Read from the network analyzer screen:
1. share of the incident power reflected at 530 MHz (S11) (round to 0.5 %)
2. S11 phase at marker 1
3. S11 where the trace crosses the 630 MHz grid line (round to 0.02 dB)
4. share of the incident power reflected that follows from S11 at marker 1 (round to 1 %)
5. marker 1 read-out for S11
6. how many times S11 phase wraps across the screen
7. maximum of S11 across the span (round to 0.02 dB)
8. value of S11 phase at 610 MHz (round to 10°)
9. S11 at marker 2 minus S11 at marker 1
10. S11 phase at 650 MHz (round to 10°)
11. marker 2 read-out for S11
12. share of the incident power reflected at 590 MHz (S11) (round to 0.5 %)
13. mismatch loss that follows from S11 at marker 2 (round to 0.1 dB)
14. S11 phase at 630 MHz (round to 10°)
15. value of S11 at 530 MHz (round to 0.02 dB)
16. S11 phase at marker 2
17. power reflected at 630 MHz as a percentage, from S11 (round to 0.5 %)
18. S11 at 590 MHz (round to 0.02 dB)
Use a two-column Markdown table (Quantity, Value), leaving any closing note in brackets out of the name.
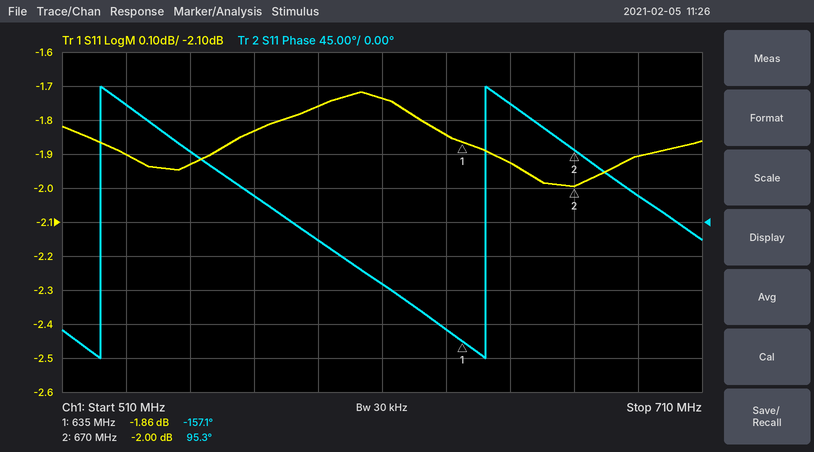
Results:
| Quantity | Value |
|---|---|
| share of the incident power reflected at 530 MHz (S11) | 64.5 % |
| S11 phase at marker 1 | -157.1° |
| S11 where the trace crosses the 630 MHz grid line | -1.84 dB |
| share of the incident power reflected that follows from S11 at marker 1 | 65 % |
| marker 1 read-out for S11 | -1.86 dB |
| how many times S11 phase wraps across the screen | 2 |
| maximum of S11 across the span | -1.72 dB |
| value of S11 phase at 610 MHz | -80° |
| S11 at marker 2 minus S11 at marker 1 | -0.14 dB |
| S11 phase at 650 MHz | 160° |
| marker 2 read-out for S11 | -2.00 dB |
| share of the incident power reflected at 590 MHz (S11) | 66.5 % |
| mismatch loss that follows from S11 at marker 2 | 4.3 dB |
| S11 phase at 630 MHz | -140° |
| value of S11 at 530 MHz | -1.90 dB |
| S11 phase at marker 2 | 95.3° |
| power reflected at 630 MHz as a percentage, from S11 | 65.5 % |
| S11 at 590 MHz | -1.76 dB |
